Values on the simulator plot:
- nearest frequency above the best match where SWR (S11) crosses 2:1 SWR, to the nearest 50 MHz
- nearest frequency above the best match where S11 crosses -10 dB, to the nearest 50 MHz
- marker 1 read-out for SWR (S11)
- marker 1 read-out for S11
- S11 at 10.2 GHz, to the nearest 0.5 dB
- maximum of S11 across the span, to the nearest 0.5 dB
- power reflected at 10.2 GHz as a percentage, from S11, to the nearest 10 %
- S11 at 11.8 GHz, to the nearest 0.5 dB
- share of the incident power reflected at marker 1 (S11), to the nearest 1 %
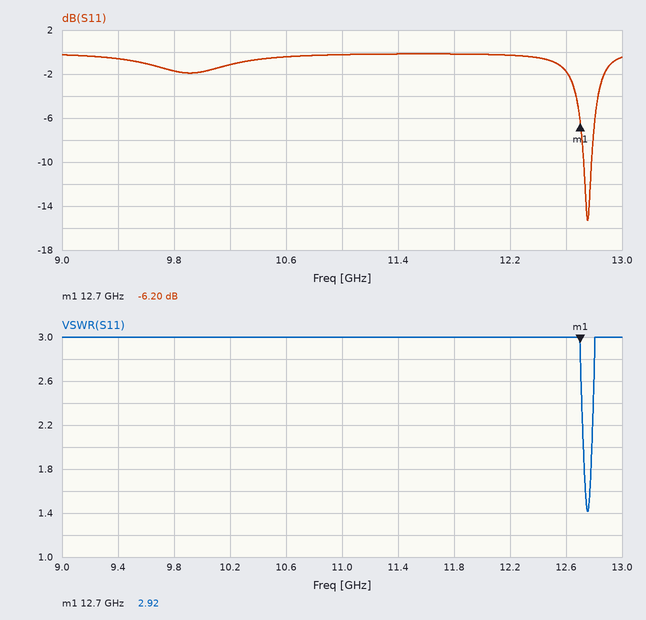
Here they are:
12.80 GHz
12.80 GHz
2.92
-6.20 dB
-1.0 dB
0.0 dB
80 %
0.0 dB
24 %
